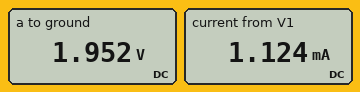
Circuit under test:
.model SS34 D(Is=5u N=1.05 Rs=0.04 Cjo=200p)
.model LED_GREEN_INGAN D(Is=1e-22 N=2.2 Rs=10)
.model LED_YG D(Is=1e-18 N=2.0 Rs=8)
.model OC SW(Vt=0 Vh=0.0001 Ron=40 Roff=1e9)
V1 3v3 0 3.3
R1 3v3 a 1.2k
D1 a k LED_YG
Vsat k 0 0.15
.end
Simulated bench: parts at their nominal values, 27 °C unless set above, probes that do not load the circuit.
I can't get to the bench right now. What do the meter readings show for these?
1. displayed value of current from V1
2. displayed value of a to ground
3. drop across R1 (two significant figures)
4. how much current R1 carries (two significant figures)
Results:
1.124 mA
1.952 V
1.3 V
1.1 mA
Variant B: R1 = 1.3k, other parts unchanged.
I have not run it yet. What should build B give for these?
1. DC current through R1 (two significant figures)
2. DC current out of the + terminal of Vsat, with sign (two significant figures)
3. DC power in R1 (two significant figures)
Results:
1.0 mA
-1.0 mA
1.4 mW
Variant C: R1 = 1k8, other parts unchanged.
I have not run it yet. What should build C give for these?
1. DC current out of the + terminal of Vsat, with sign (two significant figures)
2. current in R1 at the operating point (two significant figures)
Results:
-760 µA
760 µA
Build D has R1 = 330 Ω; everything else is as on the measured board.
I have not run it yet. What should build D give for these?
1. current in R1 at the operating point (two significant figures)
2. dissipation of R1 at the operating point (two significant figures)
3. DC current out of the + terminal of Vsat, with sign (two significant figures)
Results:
3.8 mA
4.8 mW
-3.8 mA
